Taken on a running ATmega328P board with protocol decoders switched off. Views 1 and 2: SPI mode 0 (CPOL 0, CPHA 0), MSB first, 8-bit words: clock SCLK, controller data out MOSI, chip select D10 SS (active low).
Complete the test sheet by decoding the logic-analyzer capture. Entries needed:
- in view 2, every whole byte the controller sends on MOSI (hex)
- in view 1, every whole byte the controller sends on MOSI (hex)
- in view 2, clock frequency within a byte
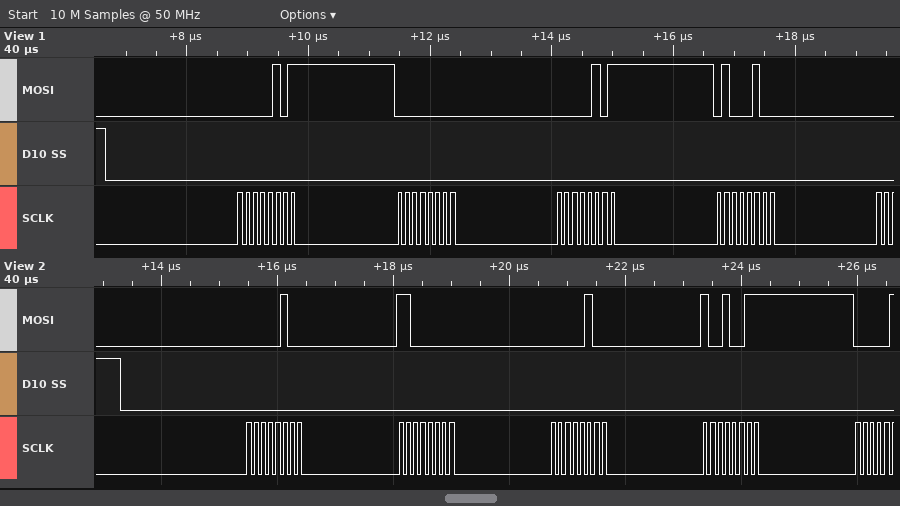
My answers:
04 C0 04 93
0x05 0x00 0x05 0x44
8 MHz
